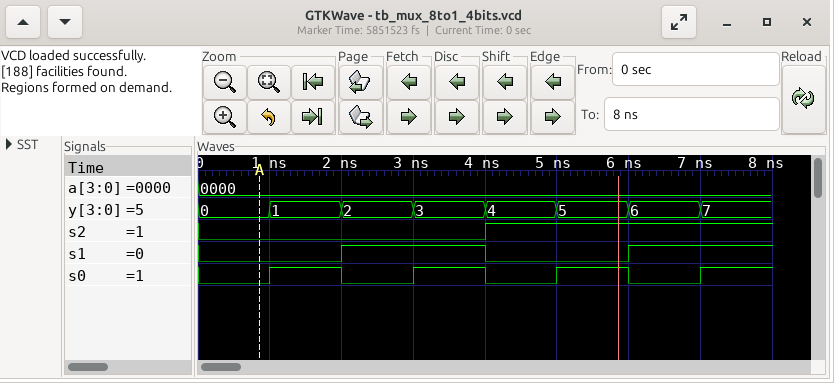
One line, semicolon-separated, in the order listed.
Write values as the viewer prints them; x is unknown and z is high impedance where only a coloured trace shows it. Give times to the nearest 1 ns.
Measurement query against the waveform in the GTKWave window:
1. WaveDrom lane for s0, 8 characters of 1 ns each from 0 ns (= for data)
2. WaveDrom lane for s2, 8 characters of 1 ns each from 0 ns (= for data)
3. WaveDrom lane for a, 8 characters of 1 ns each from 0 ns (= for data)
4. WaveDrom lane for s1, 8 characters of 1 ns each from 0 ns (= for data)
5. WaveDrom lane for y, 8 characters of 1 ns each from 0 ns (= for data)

{name: 's0', wave: '01010101'}; {name: 's2', wave: '0...1...'}; {name: 'a', wave: '=.......', data: '0000'}; {name: 's1', wave: '0.1.0.1.'}; {name: 'y', wave: '========', data: '0 1 2 3 4 5 6 7'}
